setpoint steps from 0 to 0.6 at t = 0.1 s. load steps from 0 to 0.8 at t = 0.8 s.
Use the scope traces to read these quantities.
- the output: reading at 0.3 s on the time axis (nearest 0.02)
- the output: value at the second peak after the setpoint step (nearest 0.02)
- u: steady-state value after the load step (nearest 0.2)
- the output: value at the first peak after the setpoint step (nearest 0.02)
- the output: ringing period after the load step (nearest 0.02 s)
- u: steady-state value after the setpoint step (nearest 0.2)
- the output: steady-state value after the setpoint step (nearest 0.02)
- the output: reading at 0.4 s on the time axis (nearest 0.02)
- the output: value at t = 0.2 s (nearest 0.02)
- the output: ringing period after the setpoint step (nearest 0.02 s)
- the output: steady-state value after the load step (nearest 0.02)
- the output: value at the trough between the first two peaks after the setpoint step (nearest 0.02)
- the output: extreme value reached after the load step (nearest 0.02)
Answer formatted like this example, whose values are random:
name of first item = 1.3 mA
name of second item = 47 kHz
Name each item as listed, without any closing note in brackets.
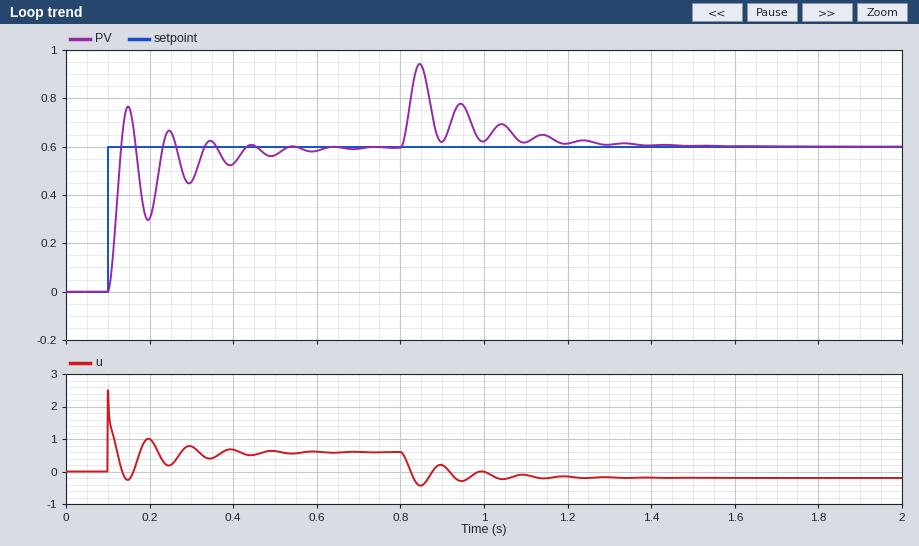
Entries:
the output: reading at 0.3 s on the time axis = 0.46
the output: value at the second peak after the setpoint step = 0.66
u: steady-state value after the load step = -0.2
the output: value at the first peak after the setpoint step = 0.76
the output: ringing period after the load step = 0.10 s
u: steady-state value after the setpoint step = 0.6
the output: steady-state value after the setpoint step = 0.60
the output: reading at 0.4 s on the time axis = 0.52
the output: value at t = 0.2 s = 0.30
the output: ringing period after the setpoint step = 0.10 s
the output: steady-state value after the load step = 0.60
the output: value at the trough between the first two peaks after the setpoint step = 0.30
the output: extreme value reached after the load step = 0.94
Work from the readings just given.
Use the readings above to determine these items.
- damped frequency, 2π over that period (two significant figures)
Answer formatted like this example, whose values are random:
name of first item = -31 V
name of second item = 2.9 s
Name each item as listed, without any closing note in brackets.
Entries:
damped frequency, 2π over that period = 63 rad/s
